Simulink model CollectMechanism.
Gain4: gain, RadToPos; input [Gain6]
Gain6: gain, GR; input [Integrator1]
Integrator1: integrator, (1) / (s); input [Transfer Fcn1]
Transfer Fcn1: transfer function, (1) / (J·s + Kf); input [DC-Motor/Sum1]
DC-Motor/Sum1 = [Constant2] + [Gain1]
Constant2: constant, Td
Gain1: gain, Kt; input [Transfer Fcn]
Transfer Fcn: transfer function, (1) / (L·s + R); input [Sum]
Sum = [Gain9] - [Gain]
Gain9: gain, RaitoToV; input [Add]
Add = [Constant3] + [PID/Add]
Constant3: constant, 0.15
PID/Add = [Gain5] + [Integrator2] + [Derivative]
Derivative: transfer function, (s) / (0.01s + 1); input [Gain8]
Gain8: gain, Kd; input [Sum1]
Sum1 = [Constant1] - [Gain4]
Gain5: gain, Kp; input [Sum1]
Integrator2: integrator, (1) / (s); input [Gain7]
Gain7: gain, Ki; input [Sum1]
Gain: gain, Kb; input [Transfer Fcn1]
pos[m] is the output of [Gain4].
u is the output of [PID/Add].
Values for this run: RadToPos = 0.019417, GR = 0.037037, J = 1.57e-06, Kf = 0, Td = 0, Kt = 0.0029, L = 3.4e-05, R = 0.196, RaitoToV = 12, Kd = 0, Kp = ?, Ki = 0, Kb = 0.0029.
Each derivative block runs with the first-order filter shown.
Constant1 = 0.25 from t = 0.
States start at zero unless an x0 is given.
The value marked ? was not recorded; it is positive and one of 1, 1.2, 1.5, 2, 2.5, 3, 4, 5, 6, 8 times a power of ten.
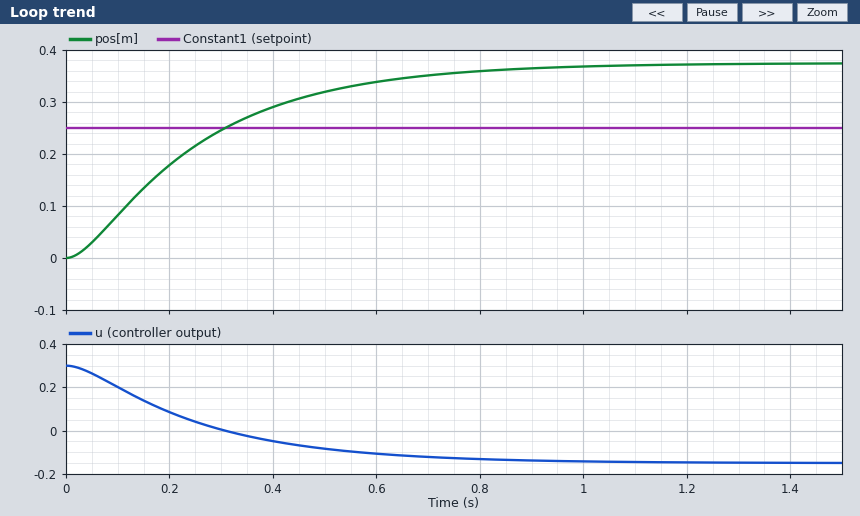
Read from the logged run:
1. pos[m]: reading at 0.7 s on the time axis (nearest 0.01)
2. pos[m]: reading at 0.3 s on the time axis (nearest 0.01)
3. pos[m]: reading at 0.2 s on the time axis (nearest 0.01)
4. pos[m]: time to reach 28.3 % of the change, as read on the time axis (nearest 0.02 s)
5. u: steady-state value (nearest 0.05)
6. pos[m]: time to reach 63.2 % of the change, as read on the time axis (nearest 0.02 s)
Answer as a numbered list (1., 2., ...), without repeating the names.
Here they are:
1. 0.35
2. 0.25
3. 0.18
4. 0.12 s
5. -0.15
6. 0.28 s
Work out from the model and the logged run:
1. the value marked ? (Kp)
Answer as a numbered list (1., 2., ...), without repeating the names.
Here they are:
1. 1.2
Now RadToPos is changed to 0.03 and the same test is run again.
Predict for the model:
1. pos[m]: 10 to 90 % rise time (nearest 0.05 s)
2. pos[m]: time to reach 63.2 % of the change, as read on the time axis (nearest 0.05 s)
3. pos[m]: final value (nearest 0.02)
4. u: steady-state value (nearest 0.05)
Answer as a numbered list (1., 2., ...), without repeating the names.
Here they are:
1. 0.30 s
2. 0.20 s
3. 0.38
4. -0.15
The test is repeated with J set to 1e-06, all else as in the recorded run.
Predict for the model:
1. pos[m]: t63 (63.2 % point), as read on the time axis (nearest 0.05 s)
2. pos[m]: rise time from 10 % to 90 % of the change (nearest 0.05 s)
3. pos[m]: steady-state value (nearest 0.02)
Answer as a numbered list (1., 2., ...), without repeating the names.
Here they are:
1. 0.30 s
2. 0.55 s
3. 0.38
